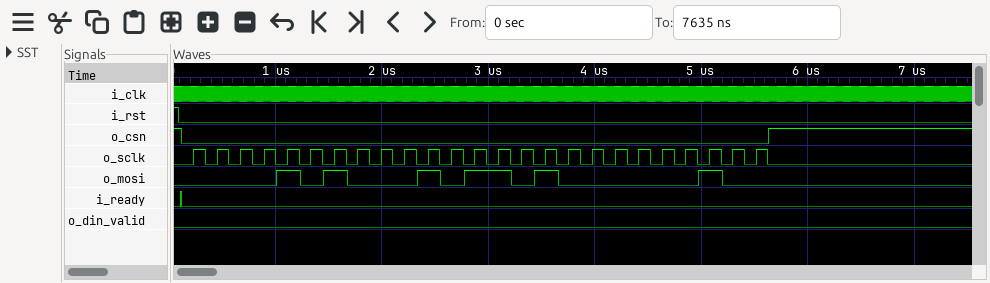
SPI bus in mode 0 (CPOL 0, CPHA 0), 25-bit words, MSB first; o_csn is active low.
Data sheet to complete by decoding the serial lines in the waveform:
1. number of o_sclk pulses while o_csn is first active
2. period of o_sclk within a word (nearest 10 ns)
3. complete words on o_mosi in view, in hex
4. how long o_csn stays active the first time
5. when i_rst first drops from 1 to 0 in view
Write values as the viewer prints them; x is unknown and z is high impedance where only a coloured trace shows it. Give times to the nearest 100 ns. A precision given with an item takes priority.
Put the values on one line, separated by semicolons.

25; 220 ns; 0145A04; 5500 ns; 100 ns
